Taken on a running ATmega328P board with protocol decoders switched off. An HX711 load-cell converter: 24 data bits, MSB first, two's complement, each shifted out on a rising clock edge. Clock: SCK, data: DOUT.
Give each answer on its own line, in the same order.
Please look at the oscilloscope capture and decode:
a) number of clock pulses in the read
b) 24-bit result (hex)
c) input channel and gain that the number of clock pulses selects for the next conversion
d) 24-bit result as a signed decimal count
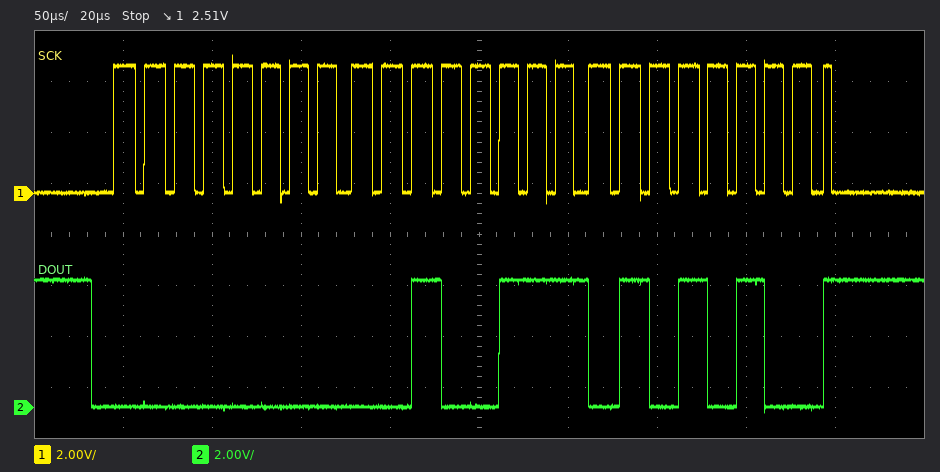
25
0x002754
channel A, gain 128
10068
